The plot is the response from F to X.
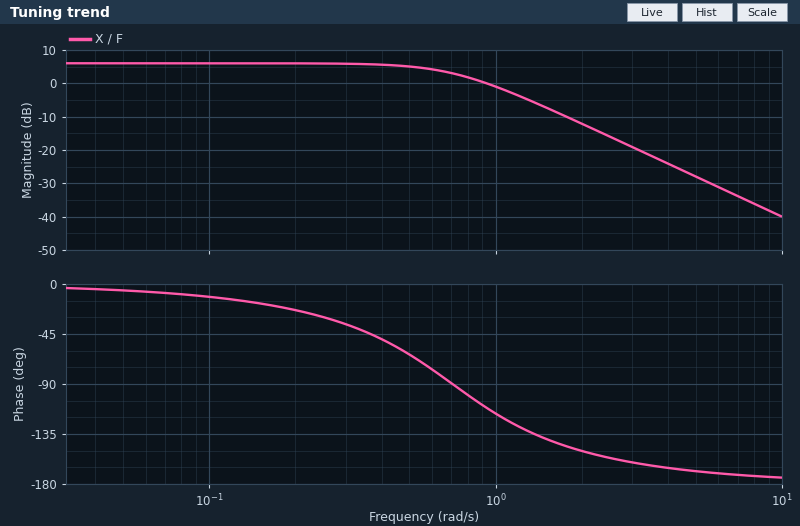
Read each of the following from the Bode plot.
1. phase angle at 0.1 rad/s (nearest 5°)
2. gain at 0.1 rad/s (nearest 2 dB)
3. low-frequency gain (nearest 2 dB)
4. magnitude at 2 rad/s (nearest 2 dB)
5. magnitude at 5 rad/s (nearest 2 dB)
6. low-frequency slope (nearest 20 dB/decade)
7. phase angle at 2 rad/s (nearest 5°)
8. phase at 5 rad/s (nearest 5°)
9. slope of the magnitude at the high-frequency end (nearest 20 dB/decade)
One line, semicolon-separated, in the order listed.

-10°; 6 dB; 6 dB; -12 dB; -28 dB; 0 dB/decade; -150°; -170°; -40 dB/decade
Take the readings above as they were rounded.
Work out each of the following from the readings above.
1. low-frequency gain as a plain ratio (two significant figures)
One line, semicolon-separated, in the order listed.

2.0
